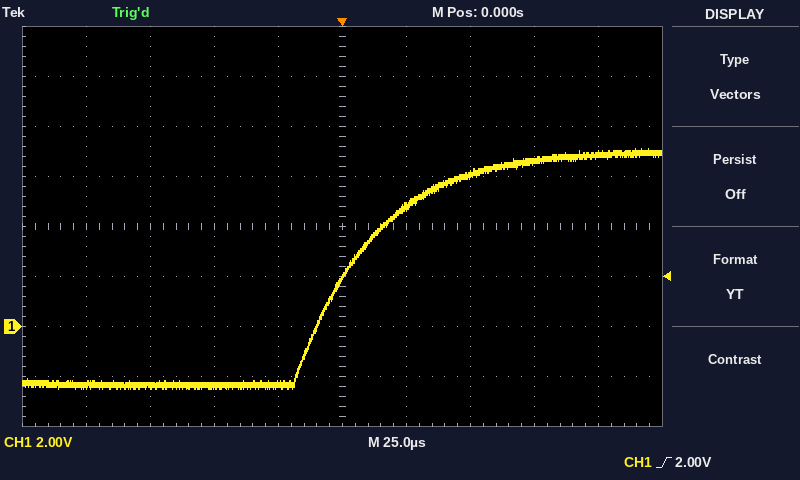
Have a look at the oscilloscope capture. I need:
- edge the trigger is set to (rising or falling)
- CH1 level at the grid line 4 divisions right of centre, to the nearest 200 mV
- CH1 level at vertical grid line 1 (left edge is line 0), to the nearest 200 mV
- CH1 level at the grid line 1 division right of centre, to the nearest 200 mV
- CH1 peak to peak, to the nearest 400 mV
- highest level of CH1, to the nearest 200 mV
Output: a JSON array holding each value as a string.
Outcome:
["rising", "6.8 V", "-2.4 V", "4.8 V", "9.6 V", "7.2 V"]
